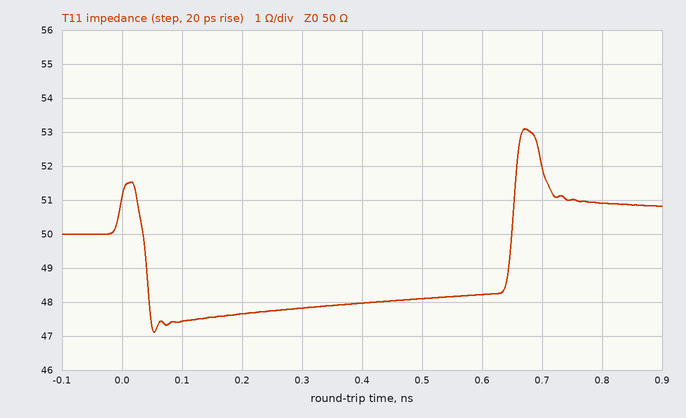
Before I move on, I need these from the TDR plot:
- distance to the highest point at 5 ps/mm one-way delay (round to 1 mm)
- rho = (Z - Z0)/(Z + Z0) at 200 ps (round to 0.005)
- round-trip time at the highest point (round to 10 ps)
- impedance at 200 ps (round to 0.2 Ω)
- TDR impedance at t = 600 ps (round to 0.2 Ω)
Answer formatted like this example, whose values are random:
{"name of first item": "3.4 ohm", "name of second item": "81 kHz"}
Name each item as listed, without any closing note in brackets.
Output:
{"distance to the highest point at 5 ps/mm one-way delay": "67 mm", "rho = (Z - Z0)/(Z + Z0) at 200 ps": "-0.025", "round-trip time at the highest point": "670 ps", "impedance at 200 ps": "47.6 Ω", "TDR impedance at t = 600 ps": "48.2 Ω"}
